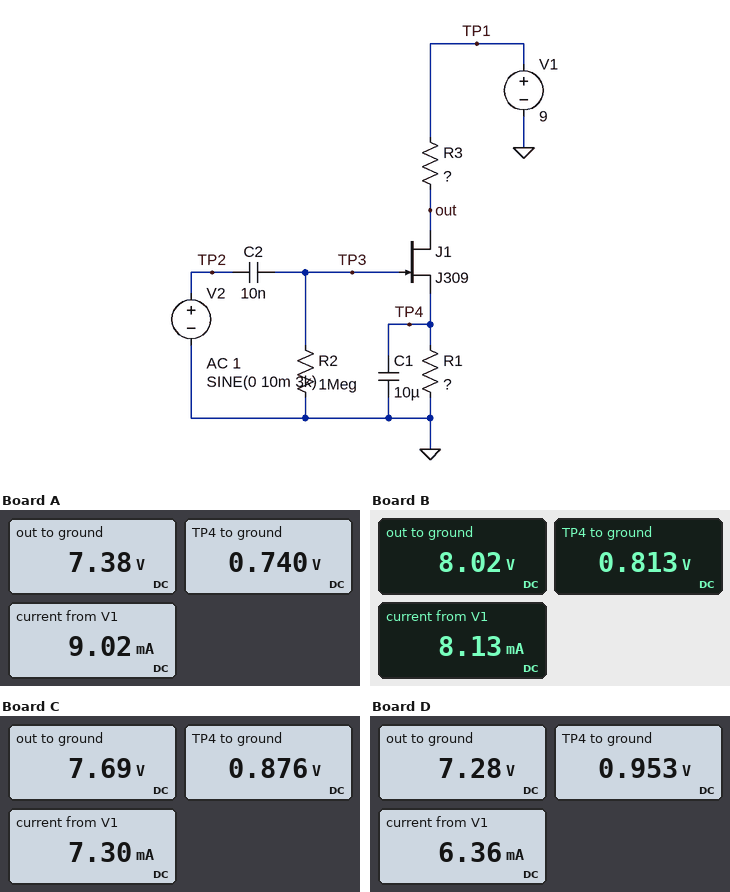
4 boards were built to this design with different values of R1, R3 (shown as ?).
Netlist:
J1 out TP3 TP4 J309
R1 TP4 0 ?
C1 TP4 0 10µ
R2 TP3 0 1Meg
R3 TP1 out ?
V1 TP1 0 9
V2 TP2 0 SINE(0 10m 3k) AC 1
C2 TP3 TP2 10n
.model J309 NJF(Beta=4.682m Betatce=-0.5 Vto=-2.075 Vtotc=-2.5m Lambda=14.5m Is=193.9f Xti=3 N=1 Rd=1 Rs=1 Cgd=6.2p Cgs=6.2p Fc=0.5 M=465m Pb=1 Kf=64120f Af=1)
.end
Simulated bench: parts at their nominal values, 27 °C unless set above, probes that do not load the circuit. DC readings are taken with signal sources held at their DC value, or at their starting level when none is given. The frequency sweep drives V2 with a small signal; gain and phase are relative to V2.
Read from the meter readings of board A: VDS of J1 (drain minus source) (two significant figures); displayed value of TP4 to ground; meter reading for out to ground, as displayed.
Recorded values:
6.6 V
0.740 V
7.38 V
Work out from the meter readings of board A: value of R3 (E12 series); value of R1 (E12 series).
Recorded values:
180 Ω
82 Ω
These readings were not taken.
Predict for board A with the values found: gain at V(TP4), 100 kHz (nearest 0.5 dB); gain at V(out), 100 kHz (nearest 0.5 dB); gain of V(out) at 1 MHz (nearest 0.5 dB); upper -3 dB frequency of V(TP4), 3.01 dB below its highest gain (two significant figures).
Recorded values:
-53.5 dB
7.5 dB
7.5 dB
440 Hz
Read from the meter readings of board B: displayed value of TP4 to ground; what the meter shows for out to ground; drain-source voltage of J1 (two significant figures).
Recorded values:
0.813 V
8.02 V
7.2 V
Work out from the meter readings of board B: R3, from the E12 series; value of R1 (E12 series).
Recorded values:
120 Ω
100 Ω
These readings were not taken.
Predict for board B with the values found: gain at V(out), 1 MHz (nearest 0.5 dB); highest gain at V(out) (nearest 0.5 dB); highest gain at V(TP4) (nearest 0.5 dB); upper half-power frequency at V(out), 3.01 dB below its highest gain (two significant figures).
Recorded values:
3.5 dB
3.5 dB
-5.5 dB
2.1 GHz
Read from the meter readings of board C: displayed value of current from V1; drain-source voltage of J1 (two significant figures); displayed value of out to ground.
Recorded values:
7.30 mA
6.8 V
7.69 V
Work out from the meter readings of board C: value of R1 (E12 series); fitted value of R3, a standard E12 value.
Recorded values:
120 Ω
180 Ω
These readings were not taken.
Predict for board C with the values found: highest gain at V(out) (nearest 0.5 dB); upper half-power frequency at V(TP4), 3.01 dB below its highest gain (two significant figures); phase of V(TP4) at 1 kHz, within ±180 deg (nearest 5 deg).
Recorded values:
6.5 dB
350 Hz
-70 deg
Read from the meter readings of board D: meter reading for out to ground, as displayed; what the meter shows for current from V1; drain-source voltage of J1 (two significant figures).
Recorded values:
7.28 V
6.36 mA
6.3 V
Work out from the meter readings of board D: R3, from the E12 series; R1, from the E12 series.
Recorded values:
270 Ω
150 Ω
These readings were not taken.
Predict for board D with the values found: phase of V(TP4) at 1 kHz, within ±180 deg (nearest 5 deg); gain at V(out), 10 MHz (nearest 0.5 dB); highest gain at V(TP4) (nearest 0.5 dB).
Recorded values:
-75 deg
9.5 dB
-4.5 dB
